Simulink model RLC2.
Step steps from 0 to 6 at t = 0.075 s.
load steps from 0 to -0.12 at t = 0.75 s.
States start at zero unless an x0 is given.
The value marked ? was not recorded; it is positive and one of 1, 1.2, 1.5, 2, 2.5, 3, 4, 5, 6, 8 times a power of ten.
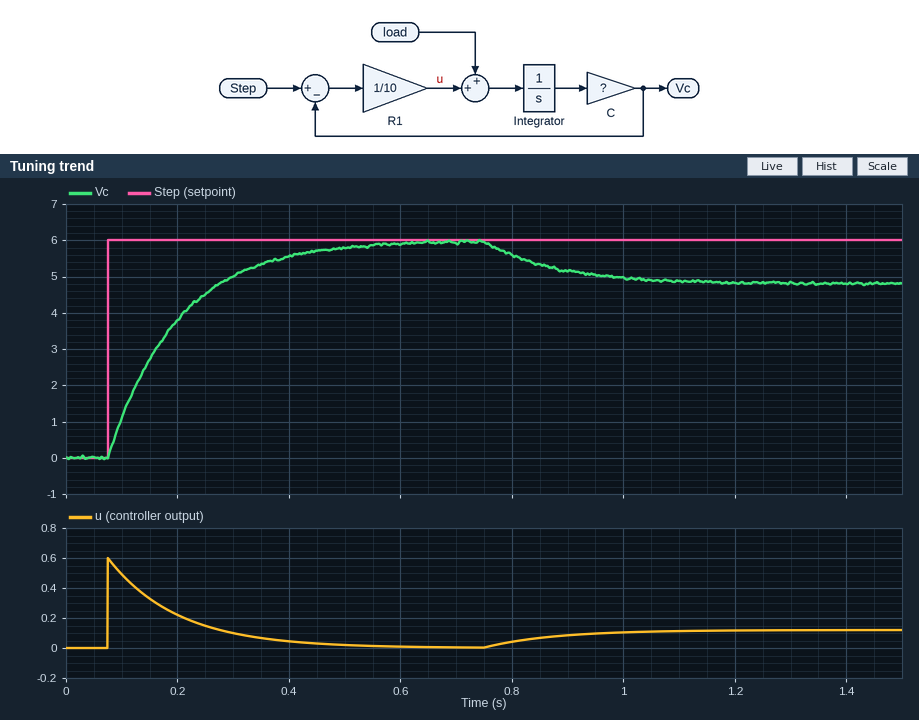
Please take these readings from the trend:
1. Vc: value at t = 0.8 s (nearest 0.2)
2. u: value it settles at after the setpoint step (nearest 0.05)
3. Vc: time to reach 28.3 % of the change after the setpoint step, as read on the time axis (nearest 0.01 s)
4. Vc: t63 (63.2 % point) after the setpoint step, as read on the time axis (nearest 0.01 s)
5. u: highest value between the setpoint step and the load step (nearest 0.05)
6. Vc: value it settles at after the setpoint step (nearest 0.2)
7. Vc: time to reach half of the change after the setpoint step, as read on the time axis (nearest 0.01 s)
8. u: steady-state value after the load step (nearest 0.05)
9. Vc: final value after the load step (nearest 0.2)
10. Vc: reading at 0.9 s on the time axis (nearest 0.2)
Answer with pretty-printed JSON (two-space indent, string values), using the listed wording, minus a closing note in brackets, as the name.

{
  "Vc: value at t = 0.8 s": "5.6",
  "u: value it settles at after the setpoint step": "0.00",
  "Vc: time to reach 28.3 % of the change after the setpoint step, as read on the time axis": "0.12 s",
  "Vc: t63 (63.2 % point) after the setpoint step, as read on the time axis": "0.20 s",
  "u: highest value between the setpoint step and the load step": "0.60",
  "Vc: value it settles at after the setpoint step": "6.0",
  "Vc: time to reach half of the change after the setpoint step, as read on the time axis": "0.16 s",
  "u: steady-state value after the load step": "0.10",
  "Vc: final value after the load step": "4.8",
  "Vc: reading at 0.9 s on the time axis": "5.2"
}
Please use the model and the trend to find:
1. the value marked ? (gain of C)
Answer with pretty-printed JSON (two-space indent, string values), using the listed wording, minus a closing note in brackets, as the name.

{
  "the value marked ?": "80"
}
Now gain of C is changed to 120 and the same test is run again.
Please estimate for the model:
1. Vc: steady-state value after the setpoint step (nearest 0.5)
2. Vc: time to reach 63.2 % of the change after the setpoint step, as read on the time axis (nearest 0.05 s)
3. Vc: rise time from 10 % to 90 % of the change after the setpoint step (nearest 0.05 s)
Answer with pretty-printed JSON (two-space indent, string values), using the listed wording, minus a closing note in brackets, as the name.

{
  "Vc: steady-state value after the setpoint step": "6.0",
  "Vc: time to reach 63.2 % of the change after the setpoint step, as read on the time axis": "0.15 s",
  "Vc: rise time from 10 % to 90 % of the change after the setpoint step": "0.20 s"
}
